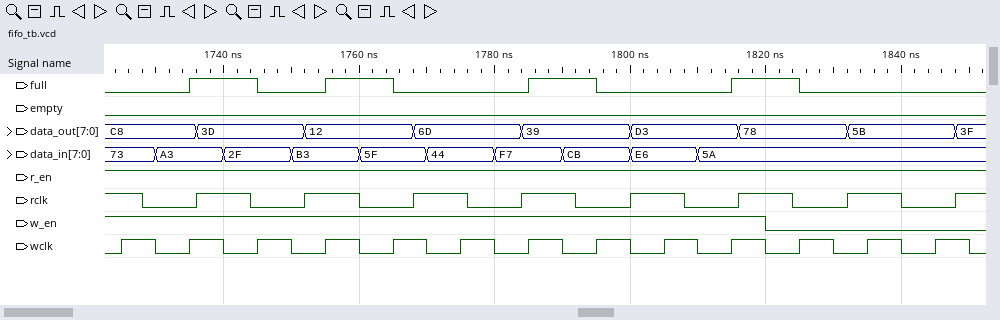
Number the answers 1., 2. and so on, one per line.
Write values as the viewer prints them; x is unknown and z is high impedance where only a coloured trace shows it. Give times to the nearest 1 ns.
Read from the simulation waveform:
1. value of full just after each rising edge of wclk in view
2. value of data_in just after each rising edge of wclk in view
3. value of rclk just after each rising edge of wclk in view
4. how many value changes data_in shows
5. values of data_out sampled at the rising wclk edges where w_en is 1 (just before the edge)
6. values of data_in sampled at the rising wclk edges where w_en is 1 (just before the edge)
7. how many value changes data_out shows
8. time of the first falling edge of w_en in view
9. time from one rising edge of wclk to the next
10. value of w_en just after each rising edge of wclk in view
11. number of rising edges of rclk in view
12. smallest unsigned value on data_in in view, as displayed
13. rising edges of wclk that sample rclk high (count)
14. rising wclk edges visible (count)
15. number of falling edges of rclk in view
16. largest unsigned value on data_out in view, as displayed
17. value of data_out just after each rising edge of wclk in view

1. 0 1 0 1 0 0 1 0 0 1 0 0 0
2. 73, A3, 2F, B3, 5F, 44, F7, CB, E6, 5A, 5A, 5A, 5A
3. 1 0 0 1 0 1 1 0 1 0 0 1 0
4. 9
5. C8, C8, 3D, 12, 12, 6D, 39, 39, D3, D3
6. 73, A3, 2F, B3, 5F, 44, F7, CB, E6, 5A
7. 8
8. 1820 ns
9. 10 ns
10. 1 1 1 1 1 1 1 1 1 1 0 0 0
11. 8
12. 2F
13. 6
14. 13
15. 8
16. D3
17. C8, C8, 3D, 12, 12, 6D, 39, 39, D3, D3, 78, 5B, 5B
